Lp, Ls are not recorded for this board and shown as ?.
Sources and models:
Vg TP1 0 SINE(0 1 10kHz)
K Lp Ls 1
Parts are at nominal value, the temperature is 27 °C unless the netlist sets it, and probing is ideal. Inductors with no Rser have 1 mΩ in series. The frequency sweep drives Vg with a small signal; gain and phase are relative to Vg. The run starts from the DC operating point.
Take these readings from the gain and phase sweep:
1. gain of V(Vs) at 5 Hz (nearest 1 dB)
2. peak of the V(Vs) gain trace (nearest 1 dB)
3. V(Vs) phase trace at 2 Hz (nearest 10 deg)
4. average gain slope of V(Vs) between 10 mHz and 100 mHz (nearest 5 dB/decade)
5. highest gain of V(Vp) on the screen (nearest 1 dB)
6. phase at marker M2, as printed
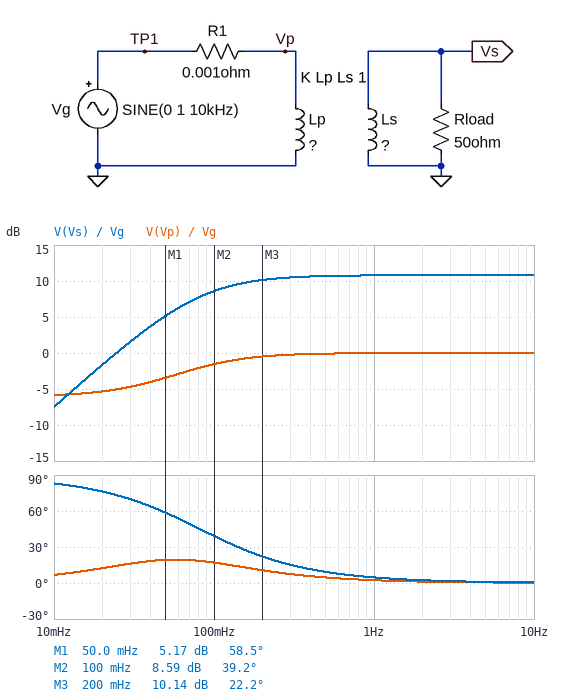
11 dB
11 dB
0 deg
15 dB/decade
0 dB
39.2 deg
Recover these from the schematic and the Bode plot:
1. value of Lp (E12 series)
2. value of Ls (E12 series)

3.9 mH
47 mH
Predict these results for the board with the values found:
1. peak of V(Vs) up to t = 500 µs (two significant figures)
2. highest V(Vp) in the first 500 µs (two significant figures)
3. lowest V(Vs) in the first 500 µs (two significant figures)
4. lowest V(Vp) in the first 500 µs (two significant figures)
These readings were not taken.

3.5 V
1.0 V
-3.5 V
-1.0 V
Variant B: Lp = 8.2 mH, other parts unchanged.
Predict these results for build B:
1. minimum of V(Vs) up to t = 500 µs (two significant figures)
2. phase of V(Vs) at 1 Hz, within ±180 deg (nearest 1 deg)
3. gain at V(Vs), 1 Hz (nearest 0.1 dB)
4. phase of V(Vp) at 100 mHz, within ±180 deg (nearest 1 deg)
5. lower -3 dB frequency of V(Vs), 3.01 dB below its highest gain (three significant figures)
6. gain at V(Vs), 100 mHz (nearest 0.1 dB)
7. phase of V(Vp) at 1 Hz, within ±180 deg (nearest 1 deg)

-2.4 V
2 deg
7.6 dB
10 deg
38.8 mHz
7.0 dB
1 deg
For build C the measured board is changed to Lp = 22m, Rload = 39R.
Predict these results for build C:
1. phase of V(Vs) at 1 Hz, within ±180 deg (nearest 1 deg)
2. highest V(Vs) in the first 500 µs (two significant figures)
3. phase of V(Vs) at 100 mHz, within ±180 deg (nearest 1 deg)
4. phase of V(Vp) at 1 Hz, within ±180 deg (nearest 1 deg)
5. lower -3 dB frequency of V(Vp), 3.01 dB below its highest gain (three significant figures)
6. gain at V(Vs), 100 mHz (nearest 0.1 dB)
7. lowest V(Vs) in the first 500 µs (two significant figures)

1 deg
1.5 V
8 deg
0 deg
10.2 mHz
3.2 dB
-1.5 V
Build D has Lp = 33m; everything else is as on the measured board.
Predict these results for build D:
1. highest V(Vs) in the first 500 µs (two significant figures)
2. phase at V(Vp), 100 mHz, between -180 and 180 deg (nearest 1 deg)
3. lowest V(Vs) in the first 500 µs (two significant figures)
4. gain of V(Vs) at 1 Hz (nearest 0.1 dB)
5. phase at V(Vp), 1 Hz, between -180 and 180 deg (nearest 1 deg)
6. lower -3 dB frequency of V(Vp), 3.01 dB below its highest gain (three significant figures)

1.2 V
3 deg
-1.2 V
1.5 dB
0 deg
6.82 mHz
